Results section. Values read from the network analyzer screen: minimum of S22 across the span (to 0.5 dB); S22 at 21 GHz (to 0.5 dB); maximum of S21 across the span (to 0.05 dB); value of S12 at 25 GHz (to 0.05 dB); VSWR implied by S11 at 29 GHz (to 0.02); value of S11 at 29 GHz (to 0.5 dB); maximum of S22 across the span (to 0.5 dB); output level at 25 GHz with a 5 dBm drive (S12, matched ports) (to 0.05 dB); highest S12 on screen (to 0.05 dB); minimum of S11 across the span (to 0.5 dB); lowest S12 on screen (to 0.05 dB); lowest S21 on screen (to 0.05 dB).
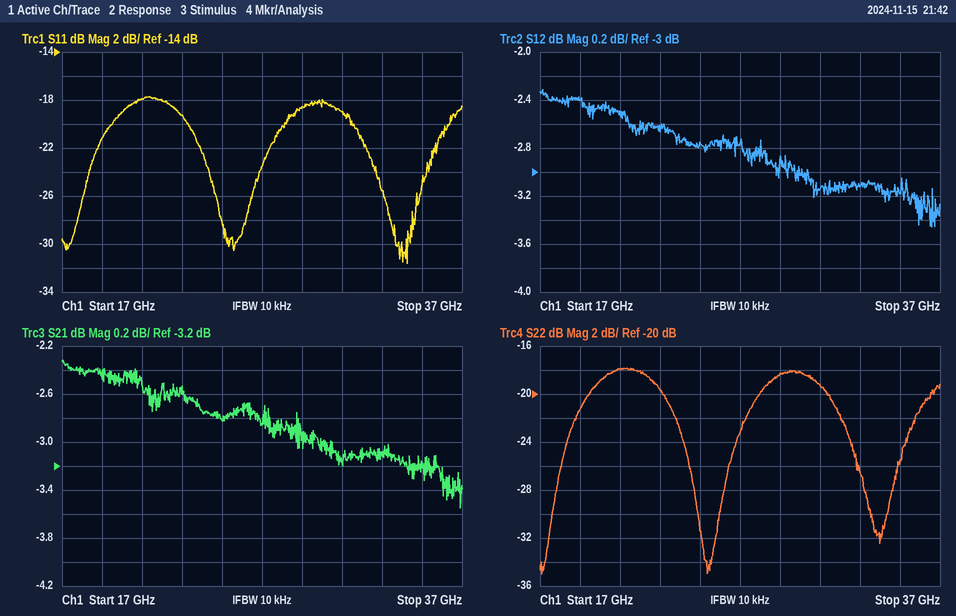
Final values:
-35.0 dB
-18.0 dB
-2.30 dB
-2.75 dB
1.26
-18.5 dB
-18.0 dB
2.25 dBm
-2.30 dB
-31.5 dB
-3.45 dB
-3.55 dB
